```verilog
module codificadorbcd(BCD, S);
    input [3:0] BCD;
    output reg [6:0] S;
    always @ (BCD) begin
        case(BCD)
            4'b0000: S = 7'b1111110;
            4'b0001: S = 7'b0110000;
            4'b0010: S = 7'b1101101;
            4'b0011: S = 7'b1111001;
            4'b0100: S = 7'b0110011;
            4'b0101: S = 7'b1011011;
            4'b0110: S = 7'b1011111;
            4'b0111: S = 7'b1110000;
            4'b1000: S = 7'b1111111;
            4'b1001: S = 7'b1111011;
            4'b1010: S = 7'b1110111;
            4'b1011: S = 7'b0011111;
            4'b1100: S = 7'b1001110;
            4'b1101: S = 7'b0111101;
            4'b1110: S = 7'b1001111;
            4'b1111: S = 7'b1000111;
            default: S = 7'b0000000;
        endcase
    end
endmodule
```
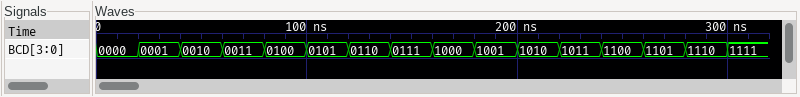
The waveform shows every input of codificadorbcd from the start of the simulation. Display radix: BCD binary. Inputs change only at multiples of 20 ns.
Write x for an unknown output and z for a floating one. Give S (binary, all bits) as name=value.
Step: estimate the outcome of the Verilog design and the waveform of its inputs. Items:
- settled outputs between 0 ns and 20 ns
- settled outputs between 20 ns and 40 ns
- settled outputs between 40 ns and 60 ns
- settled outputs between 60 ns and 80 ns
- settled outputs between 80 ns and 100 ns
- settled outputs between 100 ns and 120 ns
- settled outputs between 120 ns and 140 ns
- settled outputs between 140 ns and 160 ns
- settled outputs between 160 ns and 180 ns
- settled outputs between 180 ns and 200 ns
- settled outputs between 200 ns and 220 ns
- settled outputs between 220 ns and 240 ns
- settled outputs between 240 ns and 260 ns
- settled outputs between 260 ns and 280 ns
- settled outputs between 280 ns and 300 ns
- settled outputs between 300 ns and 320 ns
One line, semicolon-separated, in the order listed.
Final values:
S=1111110; S=0110000; S=1101101; S=1111001; S=0110011; S=1011011; S=1011111; S=1110000; S=1111111; S=1111011; S=1110111; S=0011111; S=1001110; S=0111101; S=1001111; S=1000111
